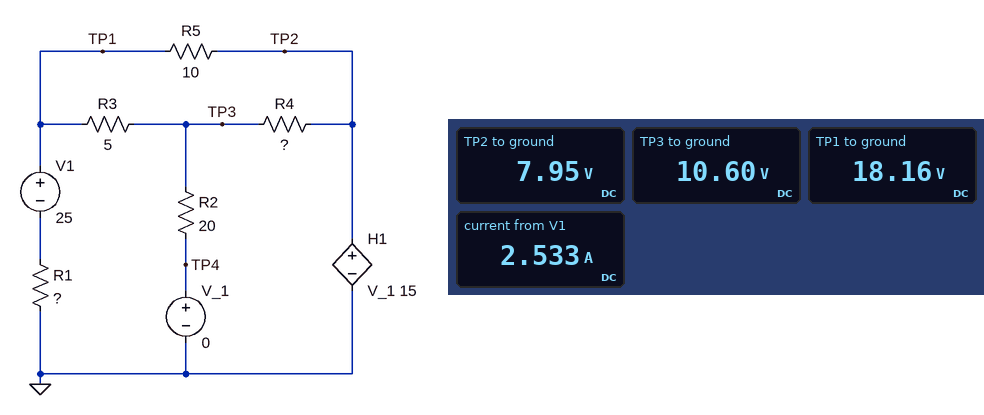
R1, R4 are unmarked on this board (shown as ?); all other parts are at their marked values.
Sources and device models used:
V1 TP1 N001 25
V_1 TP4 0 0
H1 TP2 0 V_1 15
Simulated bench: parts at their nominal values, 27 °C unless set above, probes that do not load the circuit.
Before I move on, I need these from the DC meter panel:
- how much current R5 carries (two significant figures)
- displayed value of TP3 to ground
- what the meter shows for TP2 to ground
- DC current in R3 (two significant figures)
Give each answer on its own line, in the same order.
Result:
1.0 A
10.60 V
7.95 V
1.5 A
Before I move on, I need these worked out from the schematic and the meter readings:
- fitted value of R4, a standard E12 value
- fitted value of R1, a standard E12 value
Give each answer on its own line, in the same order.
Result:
2.7 Ω
2.7 Ω
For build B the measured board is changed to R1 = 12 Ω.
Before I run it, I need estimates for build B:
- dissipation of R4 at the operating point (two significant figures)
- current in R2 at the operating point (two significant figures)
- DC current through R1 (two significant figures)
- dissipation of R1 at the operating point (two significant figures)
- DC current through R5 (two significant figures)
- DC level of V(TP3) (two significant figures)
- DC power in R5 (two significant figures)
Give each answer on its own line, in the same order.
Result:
690 mW
270 mA
1.3 A
20 W
530 mA
5.5 V
2.8 W
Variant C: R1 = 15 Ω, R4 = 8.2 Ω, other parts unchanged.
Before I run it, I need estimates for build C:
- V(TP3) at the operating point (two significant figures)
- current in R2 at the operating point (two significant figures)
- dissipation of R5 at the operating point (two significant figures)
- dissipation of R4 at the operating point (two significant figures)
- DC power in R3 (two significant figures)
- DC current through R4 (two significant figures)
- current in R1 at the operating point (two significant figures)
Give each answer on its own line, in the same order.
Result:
7.0 V
350 mA
2.1 W
370 mW
1.6 W
210 mA
1.0 A
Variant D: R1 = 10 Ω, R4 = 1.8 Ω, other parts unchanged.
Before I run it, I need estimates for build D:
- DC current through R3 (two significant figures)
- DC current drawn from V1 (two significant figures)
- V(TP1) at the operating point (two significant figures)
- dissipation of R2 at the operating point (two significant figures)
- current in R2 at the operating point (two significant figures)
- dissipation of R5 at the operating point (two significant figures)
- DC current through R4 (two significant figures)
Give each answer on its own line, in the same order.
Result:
940 mA
1.5 A
9.7 V
1.2 W
250 mA
3.5 W
690 mA
